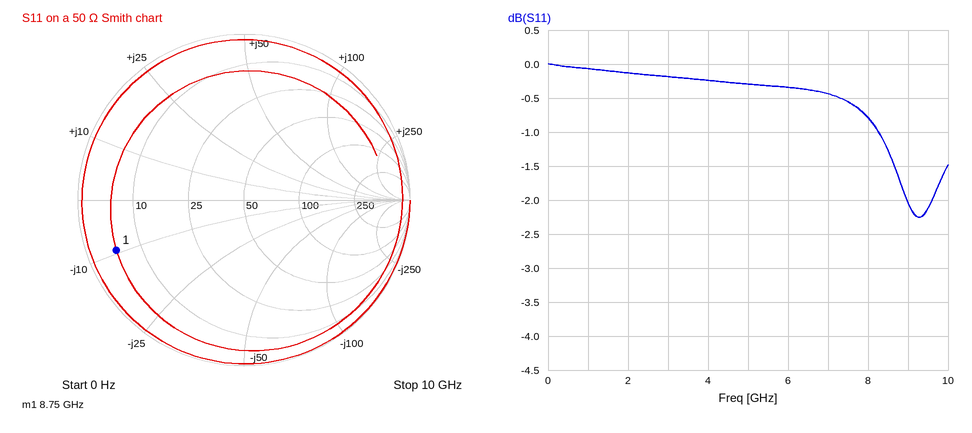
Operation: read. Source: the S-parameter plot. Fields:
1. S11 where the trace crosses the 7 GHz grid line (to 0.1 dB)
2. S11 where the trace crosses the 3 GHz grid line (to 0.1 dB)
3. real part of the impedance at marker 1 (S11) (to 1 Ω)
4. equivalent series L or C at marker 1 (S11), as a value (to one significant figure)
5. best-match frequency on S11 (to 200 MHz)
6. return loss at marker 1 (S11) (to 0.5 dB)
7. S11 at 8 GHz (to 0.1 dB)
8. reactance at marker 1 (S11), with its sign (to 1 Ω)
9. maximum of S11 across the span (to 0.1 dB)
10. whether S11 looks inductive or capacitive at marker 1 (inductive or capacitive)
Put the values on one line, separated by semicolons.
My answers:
-0.4 dB; -0.2 dB; 5 Ω; 2 pF; 9.2 GHz; 1.5 dB; -0.8 dB; -9 Ω; 0.0 dB; capacitive
